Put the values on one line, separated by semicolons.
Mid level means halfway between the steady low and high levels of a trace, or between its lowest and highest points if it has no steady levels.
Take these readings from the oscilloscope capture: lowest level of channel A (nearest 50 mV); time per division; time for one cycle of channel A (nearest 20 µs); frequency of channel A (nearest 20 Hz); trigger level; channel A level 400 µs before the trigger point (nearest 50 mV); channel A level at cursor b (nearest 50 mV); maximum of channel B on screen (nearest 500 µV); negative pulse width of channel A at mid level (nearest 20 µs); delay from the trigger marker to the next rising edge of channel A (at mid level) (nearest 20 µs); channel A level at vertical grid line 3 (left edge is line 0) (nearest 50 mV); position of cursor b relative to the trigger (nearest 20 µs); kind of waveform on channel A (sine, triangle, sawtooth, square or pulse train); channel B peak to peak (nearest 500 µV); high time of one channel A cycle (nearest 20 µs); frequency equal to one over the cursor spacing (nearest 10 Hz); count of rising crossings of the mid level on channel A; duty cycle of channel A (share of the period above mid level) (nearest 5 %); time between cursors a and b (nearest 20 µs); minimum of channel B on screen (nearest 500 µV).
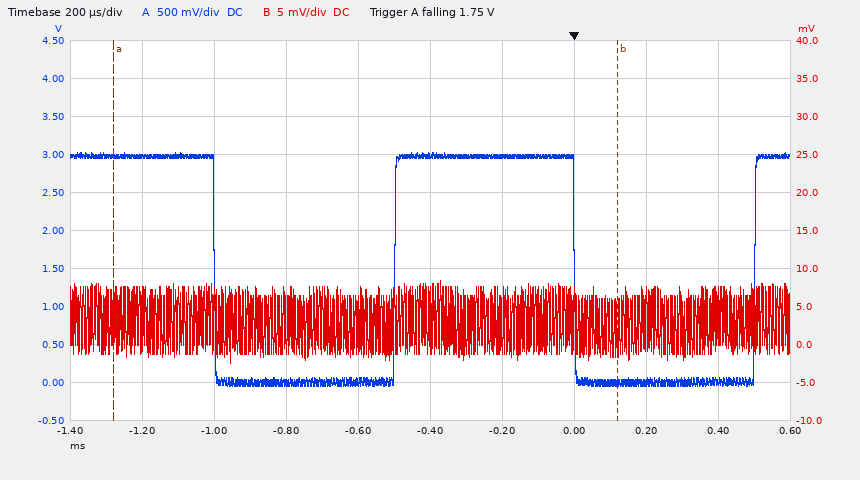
-50 mV; 200 µs; 1.00 ms; 1.00 kHz; 1.75 V; 3.00 V; 0 mV; 8.5 mV; 500 µs; 500 µs; 0 mV; +120 µs; square; 11.0 mV; 500 µs; 710 Hz; 2; 50 %; 1.40 ms; -2.5 mV
